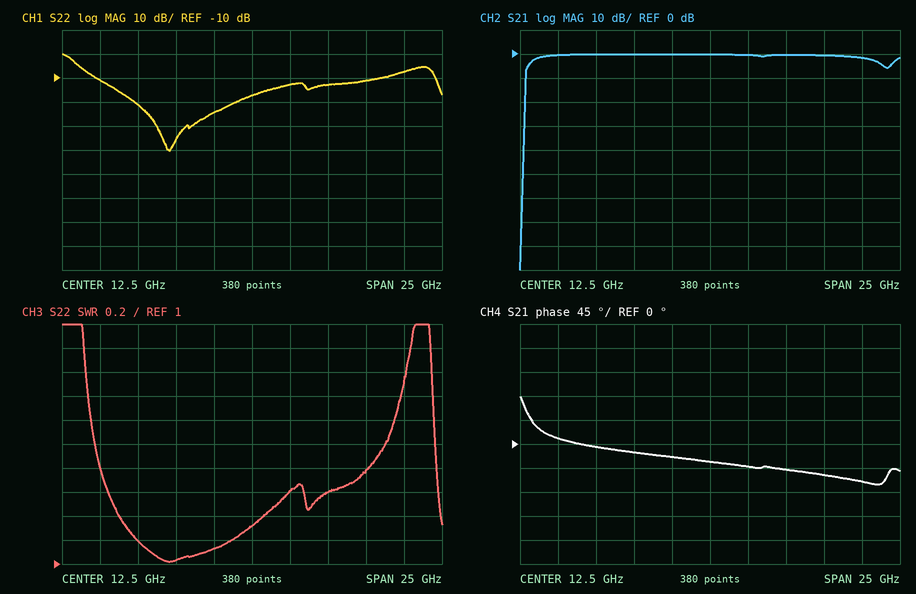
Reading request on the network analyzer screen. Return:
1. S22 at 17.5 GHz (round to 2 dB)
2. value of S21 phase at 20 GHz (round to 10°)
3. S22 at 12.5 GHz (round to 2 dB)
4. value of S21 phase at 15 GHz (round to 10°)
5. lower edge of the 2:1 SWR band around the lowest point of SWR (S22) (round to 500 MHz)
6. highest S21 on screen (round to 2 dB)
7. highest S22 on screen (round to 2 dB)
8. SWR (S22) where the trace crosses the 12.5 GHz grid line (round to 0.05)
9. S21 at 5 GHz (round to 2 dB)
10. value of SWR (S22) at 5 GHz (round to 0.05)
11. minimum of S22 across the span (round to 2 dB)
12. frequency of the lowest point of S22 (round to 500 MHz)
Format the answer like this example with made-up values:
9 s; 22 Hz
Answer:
-12 dB; -60°; -18 dB; -40°; 2.0 GHz; 0 dB; 0 dB; 1.30; 0 dB; 1.20; -40 dB; 7.0 GHz
